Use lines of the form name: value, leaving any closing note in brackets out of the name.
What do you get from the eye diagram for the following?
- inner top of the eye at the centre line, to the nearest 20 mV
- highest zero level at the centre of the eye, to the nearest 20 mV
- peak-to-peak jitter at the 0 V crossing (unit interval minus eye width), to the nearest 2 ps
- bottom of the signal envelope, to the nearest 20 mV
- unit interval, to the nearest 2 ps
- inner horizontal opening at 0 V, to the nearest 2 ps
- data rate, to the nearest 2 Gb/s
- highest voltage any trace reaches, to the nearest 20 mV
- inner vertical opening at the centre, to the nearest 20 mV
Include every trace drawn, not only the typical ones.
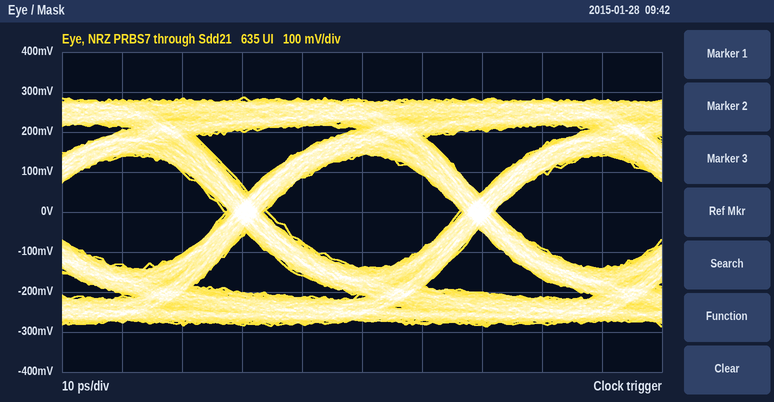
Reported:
inner top of the eye at the centre line, to the nearest 20 mV: 140 mV
highest zero level at the centre of the eye, to the nearest 20 mV: -140 mV
peak-to-peak jitter at the 0 V crossing (unit interval minus eye width), to the nearest 2 ps: 6 ps
bottom of the signal envelope, to the nearest 20 mV: -280 mV
unit interval, to the nearest 2 ps: 38 ps
inner horizontal opening at 0 V, to the nearest 2 ps: 32 ps
data rate, to the nearest 2 Gb/s: 26 Gb/s
highest voltage any trace reaches, to the nearest 20 mV: 280 mV
inner vertical opening at the centre, to the nearest 20 mV: 280 mV
